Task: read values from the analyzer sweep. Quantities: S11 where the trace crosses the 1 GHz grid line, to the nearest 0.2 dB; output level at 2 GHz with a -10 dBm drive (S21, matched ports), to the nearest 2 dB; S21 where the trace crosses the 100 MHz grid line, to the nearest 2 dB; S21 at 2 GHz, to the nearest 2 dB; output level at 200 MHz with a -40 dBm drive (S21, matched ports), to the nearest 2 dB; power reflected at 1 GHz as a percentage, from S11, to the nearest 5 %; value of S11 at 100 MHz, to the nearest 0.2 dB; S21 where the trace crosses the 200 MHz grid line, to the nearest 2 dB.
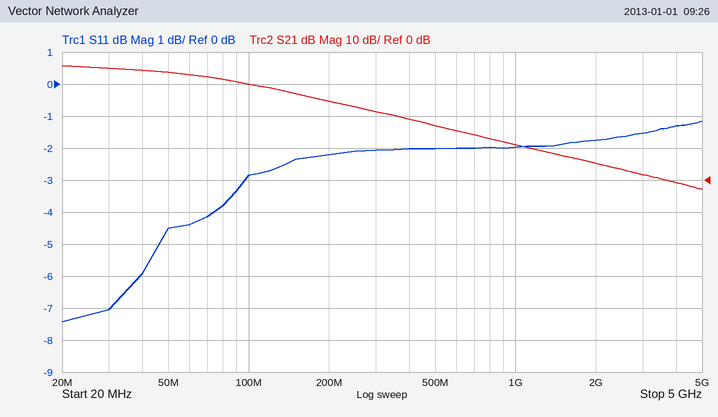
-2.0 dB
-4 dBm
30 dB
6 dB
-16 dBm
65 %
-2.8 dB
24 dB
